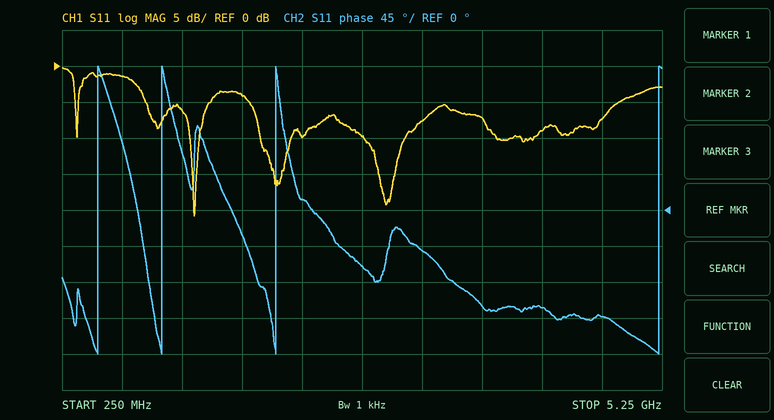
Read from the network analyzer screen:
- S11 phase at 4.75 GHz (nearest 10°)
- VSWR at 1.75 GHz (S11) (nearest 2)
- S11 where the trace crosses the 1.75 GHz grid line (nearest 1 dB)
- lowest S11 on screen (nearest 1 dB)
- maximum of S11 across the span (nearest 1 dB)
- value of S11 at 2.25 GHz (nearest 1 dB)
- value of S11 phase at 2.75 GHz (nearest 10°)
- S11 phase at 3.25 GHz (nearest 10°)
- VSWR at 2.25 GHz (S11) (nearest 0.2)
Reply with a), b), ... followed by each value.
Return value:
a) -130°
b) 4
c) -4 dB
d) -21 dB
e) 0 dB
f) -10 dB
g) -70°
h) -50°
i) 2.0
